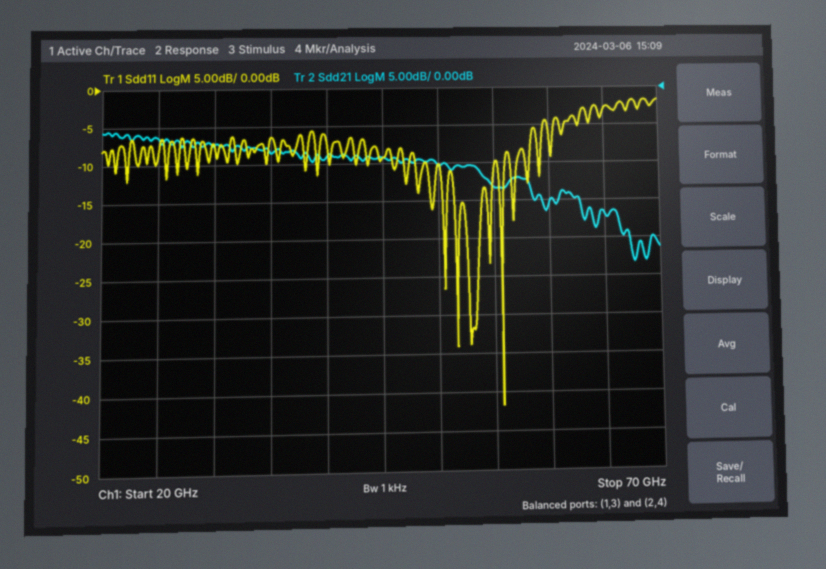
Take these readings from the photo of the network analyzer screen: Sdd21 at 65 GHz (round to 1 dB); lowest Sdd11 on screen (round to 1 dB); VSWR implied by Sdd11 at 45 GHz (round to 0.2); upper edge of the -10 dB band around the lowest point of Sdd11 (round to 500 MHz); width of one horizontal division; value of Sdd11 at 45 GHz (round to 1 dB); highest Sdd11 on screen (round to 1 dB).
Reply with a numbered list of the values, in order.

1. -17 dB
2. -42 dB
3. 2.0
4. 56.0 GHz
5. 5 GHz
6. -9 dB
7. -2 dB
